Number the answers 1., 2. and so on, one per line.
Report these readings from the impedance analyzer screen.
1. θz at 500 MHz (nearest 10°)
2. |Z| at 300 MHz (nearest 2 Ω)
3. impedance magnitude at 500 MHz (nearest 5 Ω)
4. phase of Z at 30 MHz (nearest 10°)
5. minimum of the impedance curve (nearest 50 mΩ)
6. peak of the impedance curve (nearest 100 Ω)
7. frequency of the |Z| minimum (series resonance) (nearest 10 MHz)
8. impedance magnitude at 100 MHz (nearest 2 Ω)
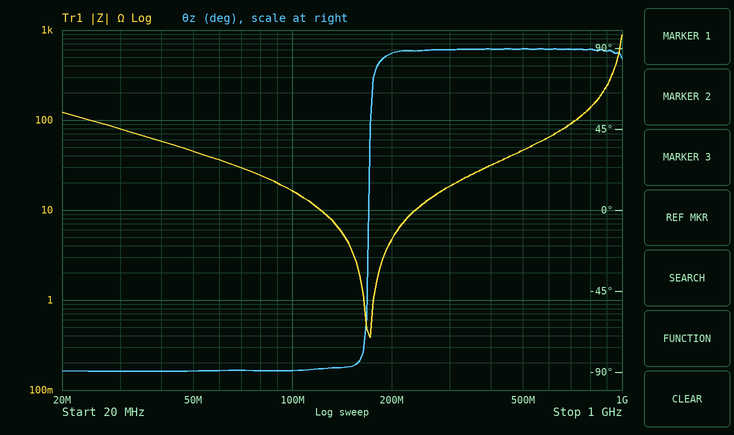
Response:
1. 90°
2. 18 Ω
3. 45 Ω
4. -90°
5. 400 mΩ
6. 900 Ω
7. 170 MHz
8. 16 Ω
